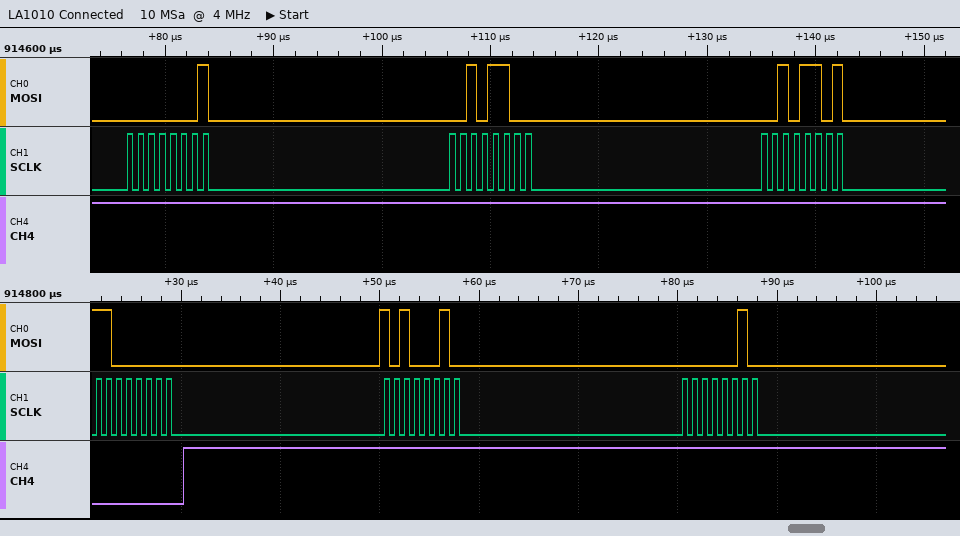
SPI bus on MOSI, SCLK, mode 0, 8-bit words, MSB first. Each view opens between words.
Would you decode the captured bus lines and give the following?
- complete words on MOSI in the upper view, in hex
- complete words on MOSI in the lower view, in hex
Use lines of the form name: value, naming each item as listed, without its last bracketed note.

complete words on MOSI in the upper view, in hex: 01, 2C, 2D
complete words on MOSI in the lower view, in hex: C0, A2, 02
